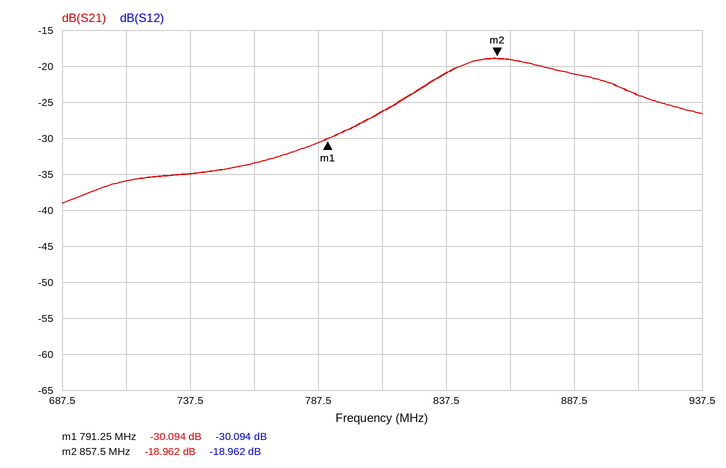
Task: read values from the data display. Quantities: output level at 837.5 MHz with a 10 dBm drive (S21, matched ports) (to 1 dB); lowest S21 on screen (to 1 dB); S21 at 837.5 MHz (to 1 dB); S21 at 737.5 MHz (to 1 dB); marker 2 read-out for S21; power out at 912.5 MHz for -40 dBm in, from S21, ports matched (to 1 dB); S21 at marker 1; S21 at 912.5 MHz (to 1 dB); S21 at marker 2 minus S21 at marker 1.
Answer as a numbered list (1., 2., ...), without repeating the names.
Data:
1. -11 dBm
2. -39 dB
3. -21 dB
4. -35 dB
5. -18.962 dB
6. -64 dBm
7. -30.094 dB
8. -24 dB
9. 11.132 dB
